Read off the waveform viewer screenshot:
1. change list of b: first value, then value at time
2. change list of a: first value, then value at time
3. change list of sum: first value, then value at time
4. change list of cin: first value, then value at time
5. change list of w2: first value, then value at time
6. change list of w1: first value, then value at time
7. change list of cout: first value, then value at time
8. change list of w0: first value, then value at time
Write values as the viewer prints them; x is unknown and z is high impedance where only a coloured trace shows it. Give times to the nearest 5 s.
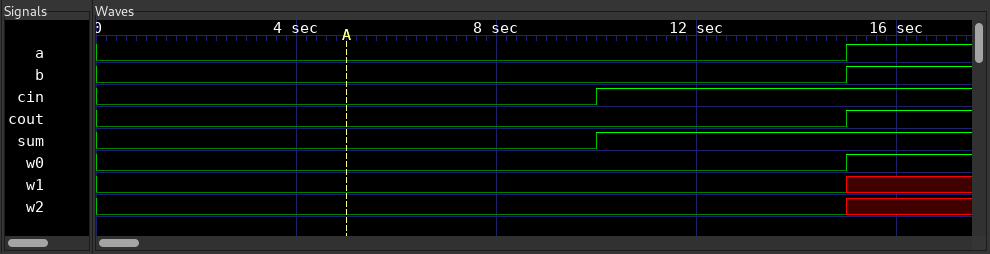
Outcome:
0, 1 at 15 s
0, 1 at 15 s
0, 1 at 10 s
0, 1 at 10 s
0, x at 15 s
0, x at 15 s
0, 1 at 15 s
0, 1 at 15 s
